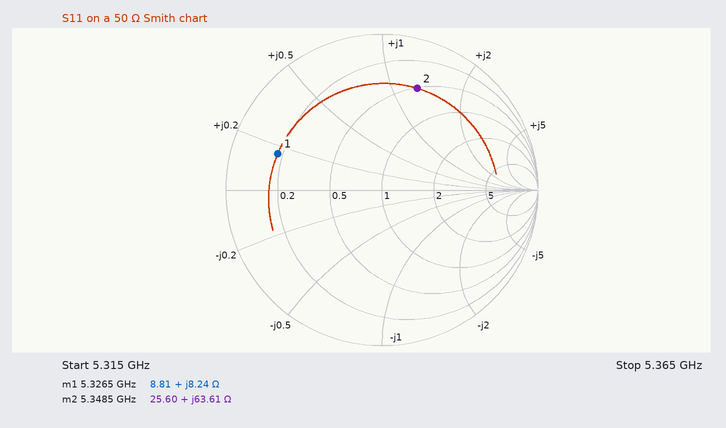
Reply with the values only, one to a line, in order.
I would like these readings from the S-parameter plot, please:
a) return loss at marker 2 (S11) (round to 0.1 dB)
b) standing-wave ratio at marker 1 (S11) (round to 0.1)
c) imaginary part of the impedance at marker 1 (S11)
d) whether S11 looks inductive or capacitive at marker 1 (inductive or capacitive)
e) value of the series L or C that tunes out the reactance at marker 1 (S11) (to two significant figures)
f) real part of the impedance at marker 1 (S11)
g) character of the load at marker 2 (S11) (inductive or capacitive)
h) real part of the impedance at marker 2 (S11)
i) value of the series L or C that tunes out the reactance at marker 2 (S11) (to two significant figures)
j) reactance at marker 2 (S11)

3.2 dB
5.8
+8.24 Ω
inductive
3.6 pF
8.81 Ω
inductive
25.60 Ω
470 fF
+63.61 Ω
